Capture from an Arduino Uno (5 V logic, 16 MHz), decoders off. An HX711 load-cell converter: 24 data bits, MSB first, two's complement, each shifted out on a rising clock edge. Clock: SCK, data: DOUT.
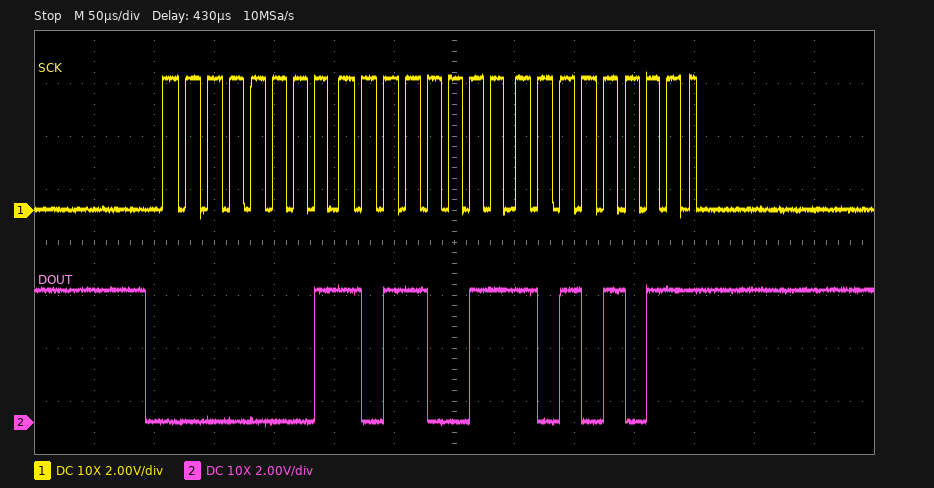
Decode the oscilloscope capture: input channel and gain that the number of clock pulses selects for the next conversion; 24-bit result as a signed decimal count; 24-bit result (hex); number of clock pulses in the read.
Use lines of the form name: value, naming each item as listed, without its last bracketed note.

input channel and gain that the number of clock pulses selects for the next conversion: channel A, gain 128
24-bit result as a signed decimal count: 111531
24-bit result: 0x01B3AB
number of clock pulses in the read: 25
